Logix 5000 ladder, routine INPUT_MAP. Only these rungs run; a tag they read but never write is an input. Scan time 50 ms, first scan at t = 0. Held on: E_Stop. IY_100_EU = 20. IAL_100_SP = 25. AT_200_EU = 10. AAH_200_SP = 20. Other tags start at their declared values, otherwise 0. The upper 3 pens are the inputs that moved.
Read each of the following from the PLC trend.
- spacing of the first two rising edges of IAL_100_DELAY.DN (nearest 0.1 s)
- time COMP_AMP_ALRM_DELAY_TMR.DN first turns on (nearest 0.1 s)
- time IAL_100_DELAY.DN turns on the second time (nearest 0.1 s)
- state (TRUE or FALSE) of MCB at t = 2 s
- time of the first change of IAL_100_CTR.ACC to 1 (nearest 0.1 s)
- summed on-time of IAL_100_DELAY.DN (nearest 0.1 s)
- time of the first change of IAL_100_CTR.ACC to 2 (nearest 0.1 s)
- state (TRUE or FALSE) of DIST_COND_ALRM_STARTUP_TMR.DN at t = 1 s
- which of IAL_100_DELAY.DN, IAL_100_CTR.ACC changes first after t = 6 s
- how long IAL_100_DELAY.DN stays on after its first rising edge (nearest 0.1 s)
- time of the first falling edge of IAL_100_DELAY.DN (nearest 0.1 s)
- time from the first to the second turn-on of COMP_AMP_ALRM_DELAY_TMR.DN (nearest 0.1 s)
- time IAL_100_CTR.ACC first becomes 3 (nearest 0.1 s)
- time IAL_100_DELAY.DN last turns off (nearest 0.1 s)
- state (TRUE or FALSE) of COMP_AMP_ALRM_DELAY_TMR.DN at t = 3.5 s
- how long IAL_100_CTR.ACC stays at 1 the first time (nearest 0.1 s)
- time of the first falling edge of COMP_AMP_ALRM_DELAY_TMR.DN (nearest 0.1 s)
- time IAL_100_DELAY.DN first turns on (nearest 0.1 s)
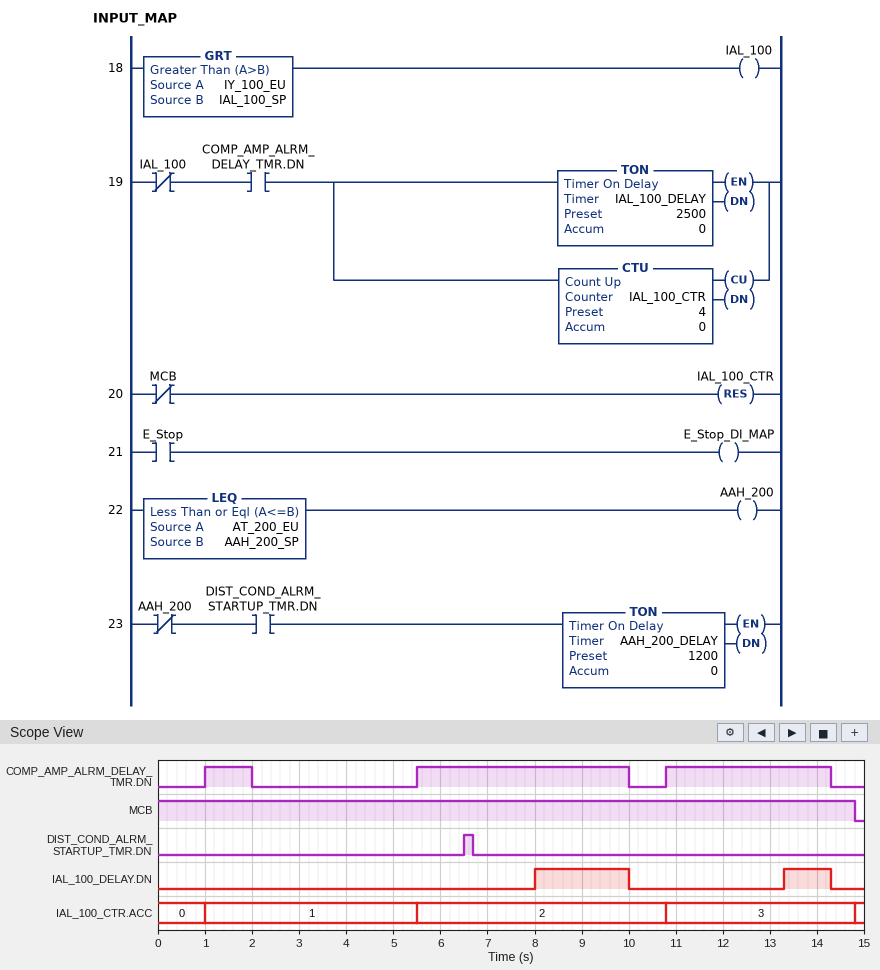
5.3 s
1.0 s
13.3 s
TRUE
1.0 s
3.0 s
5.5 s
FALSE
IAL_100_DELAY.DN
2.0 s
10.0 s
4.5 s
10.8 s
14.3 s
FALSE
4.5 s
2.0 s
8.0 s
